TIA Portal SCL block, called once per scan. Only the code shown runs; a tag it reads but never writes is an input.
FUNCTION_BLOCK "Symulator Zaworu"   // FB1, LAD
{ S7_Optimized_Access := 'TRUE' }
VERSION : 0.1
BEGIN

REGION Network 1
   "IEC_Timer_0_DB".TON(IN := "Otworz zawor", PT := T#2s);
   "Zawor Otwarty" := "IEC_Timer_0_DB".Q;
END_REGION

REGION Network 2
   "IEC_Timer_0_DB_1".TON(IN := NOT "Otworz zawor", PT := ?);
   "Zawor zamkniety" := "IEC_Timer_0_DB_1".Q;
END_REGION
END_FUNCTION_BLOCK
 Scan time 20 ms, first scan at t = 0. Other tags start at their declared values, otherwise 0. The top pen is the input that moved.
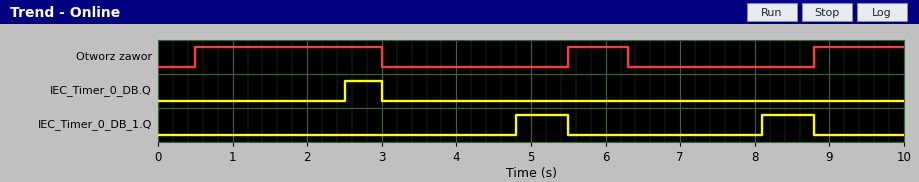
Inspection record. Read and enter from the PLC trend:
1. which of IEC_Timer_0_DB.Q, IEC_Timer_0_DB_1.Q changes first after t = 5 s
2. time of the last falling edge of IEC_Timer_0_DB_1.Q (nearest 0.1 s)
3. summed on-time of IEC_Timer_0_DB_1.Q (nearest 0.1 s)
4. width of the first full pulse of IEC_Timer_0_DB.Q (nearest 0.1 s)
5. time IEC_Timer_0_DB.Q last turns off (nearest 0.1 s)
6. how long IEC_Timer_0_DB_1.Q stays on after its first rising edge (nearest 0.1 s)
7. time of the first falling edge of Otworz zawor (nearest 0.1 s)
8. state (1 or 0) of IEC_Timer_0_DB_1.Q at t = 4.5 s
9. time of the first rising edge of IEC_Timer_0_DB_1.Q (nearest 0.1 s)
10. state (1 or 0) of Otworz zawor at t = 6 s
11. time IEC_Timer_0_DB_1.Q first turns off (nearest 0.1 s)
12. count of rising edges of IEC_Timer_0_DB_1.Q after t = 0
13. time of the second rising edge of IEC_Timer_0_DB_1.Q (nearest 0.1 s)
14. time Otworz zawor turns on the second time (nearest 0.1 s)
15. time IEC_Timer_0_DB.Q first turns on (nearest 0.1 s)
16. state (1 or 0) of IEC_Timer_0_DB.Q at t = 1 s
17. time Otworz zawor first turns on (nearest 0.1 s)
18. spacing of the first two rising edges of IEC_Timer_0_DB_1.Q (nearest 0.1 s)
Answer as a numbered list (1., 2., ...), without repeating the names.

1. IEC_Timer_0_DB_1.Q
2. 8.8 s
3. 1.4 s
4. 0.5 s
5. 3.0 s
6. 0.7 s
7. 3.0 s
8. 0
9. 4.8 s
10. 1
11. 5.5 s
12. 2
13. 8.1 s
14. 5.5 s
15. 2.5 s
16. 0
17. 0.5 s
18. 3.3 s
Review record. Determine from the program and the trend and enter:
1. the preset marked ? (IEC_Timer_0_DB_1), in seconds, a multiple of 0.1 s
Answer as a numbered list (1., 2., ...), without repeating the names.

1. 1.8 s
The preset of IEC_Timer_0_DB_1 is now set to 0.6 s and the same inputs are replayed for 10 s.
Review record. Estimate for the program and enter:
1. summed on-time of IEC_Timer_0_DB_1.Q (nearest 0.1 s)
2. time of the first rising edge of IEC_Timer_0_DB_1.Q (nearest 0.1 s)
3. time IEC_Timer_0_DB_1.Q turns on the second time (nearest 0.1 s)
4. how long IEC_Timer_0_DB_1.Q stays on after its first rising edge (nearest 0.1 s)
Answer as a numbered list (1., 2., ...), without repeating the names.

1. 3.8 s
2. 3.6 s
3. 6.9 s
4. 1.9 s
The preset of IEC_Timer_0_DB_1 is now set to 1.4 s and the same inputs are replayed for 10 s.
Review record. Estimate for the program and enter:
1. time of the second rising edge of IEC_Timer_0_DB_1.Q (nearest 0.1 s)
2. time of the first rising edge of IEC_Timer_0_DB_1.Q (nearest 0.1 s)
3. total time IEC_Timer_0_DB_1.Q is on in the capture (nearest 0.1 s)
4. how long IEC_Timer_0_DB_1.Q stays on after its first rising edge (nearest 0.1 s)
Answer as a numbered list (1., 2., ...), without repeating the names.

1. 7.7 s
2. 4.4 s
3. 2.2 s
4. 1.1 s
